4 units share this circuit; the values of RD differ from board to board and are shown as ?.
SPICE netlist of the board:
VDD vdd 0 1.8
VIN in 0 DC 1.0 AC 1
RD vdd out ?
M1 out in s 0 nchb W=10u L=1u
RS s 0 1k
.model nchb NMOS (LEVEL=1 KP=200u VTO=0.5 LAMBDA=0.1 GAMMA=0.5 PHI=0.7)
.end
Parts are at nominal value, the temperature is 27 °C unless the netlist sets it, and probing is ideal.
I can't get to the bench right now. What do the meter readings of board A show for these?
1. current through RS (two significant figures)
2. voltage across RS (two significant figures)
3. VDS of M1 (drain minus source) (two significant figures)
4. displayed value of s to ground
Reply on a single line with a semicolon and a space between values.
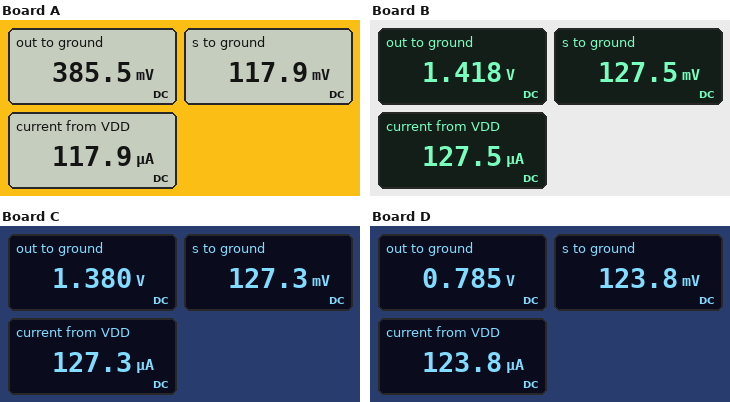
120 µA; 120 mV; 270 mV; 117.9 mV
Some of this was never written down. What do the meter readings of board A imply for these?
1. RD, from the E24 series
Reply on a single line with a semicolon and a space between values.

12 kΩ
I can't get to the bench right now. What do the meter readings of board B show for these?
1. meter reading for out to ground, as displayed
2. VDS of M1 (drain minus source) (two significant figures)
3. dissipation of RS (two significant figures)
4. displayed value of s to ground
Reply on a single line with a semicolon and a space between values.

1.418 V; 1.3 V; 16 µW; 127.5 mV
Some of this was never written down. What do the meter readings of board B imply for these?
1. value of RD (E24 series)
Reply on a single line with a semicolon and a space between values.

3 kΩ
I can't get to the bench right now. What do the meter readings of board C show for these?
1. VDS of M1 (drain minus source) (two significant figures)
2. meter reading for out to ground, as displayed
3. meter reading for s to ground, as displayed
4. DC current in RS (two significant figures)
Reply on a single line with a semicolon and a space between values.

1.3 V; 1.380 V; 127.3 mV; 130 µA
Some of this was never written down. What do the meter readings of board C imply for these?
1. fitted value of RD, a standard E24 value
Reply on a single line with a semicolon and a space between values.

3.3 kΩ
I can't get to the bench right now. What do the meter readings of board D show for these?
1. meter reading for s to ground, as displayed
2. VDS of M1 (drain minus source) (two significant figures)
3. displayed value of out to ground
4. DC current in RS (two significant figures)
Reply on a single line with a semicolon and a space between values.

123.8 mV; 660 mV; 0.785 V; 120 µA
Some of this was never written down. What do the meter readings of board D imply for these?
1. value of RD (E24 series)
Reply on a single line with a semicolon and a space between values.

8.2 kΩ
